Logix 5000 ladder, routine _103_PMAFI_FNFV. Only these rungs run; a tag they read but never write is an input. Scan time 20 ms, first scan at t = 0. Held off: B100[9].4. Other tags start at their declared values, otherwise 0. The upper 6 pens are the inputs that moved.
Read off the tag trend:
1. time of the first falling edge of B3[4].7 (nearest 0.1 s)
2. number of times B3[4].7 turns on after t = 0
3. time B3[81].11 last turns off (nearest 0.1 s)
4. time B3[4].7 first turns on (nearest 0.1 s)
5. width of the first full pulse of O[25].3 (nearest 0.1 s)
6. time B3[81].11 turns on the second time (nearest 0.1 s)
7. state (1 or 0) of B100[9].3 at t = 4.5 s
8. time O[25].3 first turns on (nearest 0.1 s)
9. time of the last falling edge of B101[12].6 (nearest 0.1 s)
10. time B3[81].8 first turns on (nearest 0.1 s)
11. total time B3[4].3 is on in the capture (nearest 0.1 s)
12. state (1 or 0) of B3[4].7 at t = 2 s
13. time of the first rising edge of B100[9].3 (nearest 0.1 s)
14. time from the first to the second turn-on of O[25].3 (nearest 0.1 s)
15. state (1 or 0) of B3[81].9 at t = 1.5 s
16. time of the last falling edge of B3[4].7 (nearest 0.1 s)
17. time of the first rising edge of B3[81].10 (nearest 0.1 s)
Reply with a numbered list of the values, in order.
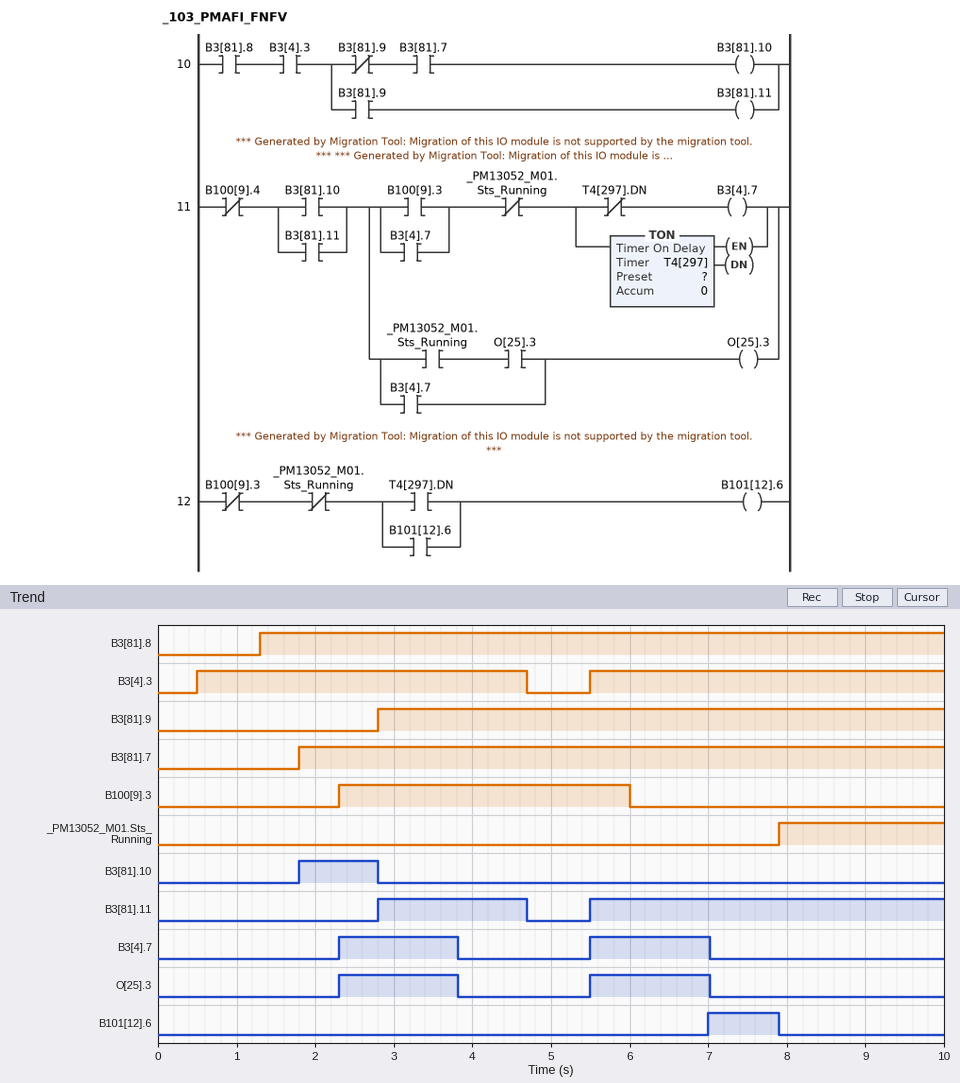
1. 3.8 s
2. 2
3. 4.7 s
4. 2.3 s
5. 1.5 s
6. 5.5 s
7. 1
8. 2.3 s
9. 7.9 s
10. 1.3 s
11. 8.7 s
12. 0
13. 2.3 s
14. 3.2 s
15. 0
16. 7.0 s
17. 1.8 s
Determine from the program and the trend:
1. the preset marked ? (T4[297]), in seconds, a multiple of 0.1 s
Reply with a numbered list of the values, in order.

1. 1.5 s
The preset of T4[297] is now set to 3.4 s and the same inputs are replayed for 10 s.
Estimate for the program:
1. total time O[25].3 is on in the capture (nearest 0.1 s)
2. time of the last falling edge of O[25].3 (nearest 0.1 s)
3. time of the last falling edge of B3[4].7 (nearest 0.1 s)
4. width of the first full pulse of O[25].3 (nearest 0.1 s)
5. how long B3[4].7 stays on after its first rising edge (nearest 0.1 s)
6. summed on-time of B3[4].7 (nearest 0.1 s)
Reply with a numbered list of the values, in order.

1. 6.9 s
2. 4.7 s
3. 7.9 s
4. 2.4 s
5. 2.4 s
6. 4.8 s
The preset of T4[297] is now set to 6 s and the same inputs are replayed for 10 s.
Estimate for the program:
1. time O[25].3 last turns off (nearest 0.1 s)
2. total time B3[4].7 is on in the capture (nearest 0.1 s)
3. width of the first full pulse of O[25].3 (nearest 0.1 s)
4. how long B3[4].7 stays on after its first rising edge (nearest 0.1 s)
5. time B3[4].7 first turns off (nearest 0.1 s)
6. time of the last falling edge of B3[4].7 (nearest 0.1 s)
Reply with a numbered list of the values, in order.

1. 4.7 s
2. 4.8 s
3. 2.4 s
4. 2.4 s
5. 4.7 s
6. 7.9 s
